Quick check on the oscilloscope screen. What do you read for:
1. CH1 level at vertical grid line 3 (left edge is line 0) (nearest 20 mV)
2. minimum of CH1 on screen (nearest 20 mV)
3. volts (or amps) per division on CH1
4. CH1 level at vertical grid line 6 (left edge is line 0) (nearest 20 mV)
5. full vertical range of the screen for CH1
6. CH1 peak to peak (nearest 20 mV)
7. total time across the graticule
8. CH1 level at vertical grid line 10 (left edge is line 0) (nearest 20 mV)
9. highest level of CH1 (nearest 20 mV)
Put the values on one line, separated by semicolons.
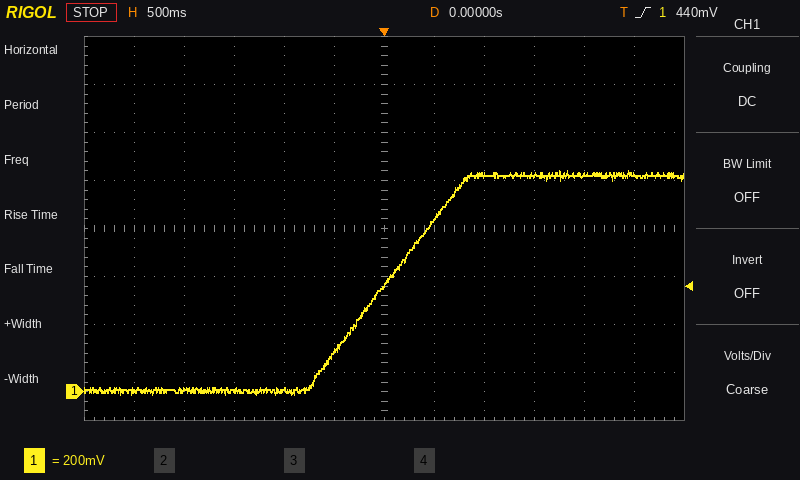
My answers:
0 mV; -20 mV; 200 mV; 440 mV; 1.6 V; 940 mV; 6 s; 900 mV; 920 mV
